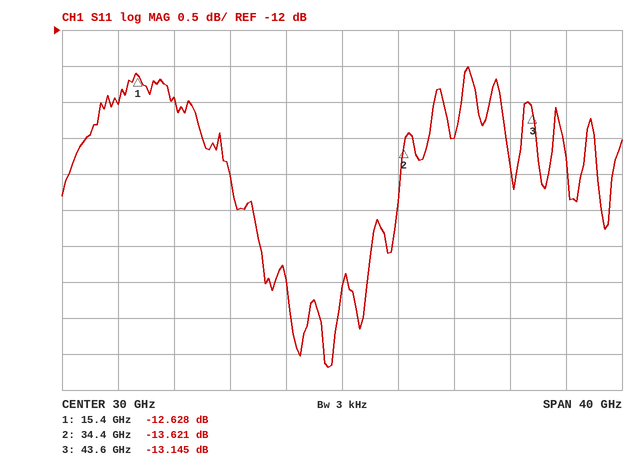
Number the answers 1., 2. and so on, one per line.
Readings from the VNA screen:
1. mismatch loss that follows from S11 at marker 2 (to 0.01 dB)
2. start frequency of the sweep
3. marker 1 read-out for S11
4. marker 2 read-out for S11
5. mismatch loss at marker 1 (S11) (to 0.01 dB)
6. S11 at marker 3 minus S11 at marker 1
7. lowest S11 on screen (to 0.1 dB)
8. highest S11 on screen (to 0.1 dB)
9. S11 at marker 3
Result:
1. 0.19 dB
2. 10 GHz
3. -12.628 dB
4. -13.621 dB
5. 0.24 dB
6. -0.517 dB
7. -16.7 dB
8. -12.5 dB
9. -13.145 dB
